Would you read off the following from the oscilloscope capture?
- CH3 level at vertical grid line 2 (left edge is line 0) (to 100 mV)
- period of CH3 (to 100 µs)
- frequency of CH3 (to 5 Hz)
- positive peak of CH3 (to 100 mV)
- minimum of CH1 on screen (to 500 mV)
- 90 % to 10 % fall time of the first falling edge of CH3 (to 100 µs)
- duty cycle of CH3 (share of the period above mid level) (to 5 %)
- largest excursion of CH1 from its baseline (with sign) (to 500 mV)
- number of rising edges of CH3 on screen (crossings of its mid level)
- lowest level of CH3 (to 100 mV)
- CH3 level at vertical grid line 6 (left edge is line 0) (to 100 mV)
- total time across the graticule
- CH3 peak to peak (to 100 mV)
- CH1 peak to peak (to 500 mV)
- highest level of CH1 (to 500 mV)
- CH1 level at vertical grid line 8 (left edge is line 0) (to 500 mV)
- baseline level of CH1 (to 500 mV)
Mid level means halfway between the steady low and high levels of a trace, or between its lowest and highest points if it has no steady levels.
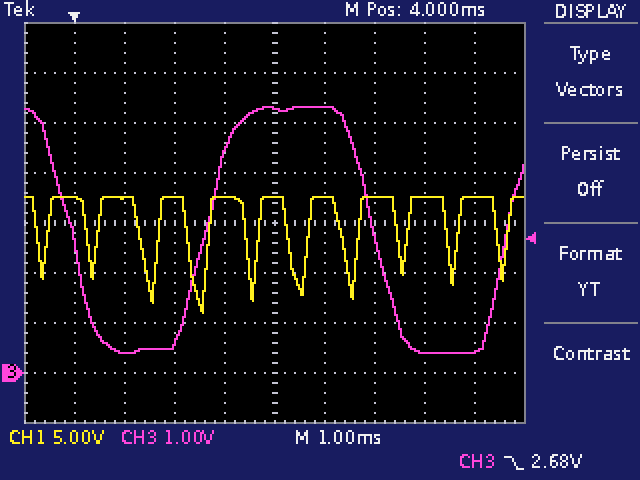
400 mV
6.0 ms
165 Hz
5.3 V
6.0 V
1.0 ms
55 %
-11.5 V
2
400 mV
5.3 V
10 ms
4.9 V
11.5 V
17.5 V
17.5 V
17.5 V
